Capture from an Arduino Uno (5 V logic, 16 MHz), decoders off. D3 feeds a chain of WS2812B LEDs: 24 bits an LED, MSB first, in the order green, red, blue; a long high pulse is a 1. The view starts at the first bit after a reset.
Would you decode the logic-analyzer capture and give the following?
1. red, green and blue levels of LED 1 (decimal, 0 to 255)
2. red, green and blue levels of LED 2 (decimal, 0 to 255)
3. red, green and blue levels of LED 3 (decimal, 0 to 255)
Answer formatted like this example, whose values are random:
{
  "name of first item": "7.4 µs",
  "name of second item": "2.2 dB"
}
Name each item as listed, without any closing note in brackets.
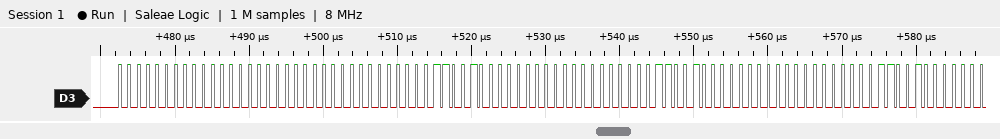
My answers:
{
  "red, green and blue levels of LED 1": "0, 0, 0",
  "red, green and blue levels of LED 2": "50, 0, 0",
  "red, green and blue levels of LED 3": "50, 0, 0"
}
